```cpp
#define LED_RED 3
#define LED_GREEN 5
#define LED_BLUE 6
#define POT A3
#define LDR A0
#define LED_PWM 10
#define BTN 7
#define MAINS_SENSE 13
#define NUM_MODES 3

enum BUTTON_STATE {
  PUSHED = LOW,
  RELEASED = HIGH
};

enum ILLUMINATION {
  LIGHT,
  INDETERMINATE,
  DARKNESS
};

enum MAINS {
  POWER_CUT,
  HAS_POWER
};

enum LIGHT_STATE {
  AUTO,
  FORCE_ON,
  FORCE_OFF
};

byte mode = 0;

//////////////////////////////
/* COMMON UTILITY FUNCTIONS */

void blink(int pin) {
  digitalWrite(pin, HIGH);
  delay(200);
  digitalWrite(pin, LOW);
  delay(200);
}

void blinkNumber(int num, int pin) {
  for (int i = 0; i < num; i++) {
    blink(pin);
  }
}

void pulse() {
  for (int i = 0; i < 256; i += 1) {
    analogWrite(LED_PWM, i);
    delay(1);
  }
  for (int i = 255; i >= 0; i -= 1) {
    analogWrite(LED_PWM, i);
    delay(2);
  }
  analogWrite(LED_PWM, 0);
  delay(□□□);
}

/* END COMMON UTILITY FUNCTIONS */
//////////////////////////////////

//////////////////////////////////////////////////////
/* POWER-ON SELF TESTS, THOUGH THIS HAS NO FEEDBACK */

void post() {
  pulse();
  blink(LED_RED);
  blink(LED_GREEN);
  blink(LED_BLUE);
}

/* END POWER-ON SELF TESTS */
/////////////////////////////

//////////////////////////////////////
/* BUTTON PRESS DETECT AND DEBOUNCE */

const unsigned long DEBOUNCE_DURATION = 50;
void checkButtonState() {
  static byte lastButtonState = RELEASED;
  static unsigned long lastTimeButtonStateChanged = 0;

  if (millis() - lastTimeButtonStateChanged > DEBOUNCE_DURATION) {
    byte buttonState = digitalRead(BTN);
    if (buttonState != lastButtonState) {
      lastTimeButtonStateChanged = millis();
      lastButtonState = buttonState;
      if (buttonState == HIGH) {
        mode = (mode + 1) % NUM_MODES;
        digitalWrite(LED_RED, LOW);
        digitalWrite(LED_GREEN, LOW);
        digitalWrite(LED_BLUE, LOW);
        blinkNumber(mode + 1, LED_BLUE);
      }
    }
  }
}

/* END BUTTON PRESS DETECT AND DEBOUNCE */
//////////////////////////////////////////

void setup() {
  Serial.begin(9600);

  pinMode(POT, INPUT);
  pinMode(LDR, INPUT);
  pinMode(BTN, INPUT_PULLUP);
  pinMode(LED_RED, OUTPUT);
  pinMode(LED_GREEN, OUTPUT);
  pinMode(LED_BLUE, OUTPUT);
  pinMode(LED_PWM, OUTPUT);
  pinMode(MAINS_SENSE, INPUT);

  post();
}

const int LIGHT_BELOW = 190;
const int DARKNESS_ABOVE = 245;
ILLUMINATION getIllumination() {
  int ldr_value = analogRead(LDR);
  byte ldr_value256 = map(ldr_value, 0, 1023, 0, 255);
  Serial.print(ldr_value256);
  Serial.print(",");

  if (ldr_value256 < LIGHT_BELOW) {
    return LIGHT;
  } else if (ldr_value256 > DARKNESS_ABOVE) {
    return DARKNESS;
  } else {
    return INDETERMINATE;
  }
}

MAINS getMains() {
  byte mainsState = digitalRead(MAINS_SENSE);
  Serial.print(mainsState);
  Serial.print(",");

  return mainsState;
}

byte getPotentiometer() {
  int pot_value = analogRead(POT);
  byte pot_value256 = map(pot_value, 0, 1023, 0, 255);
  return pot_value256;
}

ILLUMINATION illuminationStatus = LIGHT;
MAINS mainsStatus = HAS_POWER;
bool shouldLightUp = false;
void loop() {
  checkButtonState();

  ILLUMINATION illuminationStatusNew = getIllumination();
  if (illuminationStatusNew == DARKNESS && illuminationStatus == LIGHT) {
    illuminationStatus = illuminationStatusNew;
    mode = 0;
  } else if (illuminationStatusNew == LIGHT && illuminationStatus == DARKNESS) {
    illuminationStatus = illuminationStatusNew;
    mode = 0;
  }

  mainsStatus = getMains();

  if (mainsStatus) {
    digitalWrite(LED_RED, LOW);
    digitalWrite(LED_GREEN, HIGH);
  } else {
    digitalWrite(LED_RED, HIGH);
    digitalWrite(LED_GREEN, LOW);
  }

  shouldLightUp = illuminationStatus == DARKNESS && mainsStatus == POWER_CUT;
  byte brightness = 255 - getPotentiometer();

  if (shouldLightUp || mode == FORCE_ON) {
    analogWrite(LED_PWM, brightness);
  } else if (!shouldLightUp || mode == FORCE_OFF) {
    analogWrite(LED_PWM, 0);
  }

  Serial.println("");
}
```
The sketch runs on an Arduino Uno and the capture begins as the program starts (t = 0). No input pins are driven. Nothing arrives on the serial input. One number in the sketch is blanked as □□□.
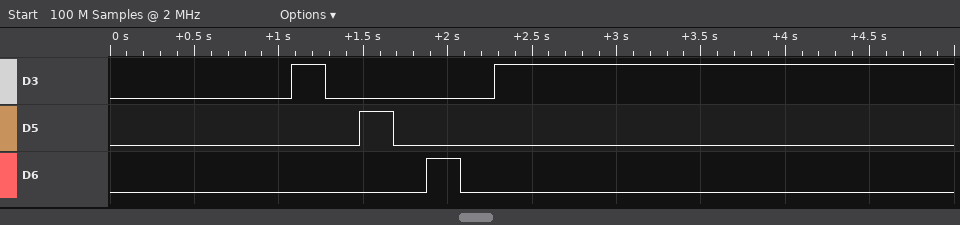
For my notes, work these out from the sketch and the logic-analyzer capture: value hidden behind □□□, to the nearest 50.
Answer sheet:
300
